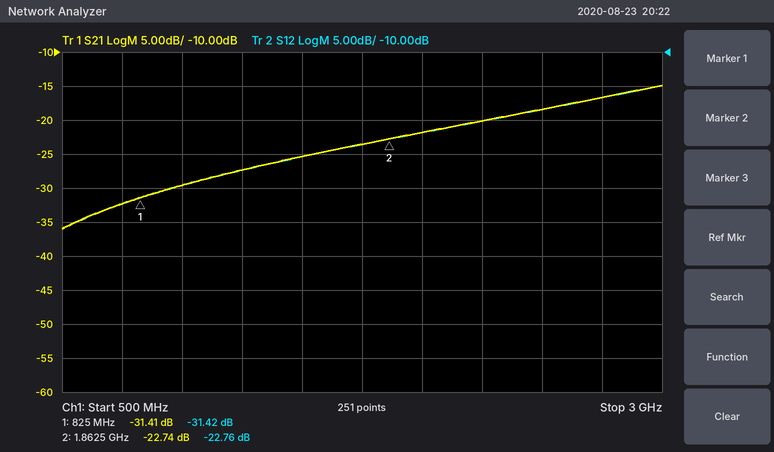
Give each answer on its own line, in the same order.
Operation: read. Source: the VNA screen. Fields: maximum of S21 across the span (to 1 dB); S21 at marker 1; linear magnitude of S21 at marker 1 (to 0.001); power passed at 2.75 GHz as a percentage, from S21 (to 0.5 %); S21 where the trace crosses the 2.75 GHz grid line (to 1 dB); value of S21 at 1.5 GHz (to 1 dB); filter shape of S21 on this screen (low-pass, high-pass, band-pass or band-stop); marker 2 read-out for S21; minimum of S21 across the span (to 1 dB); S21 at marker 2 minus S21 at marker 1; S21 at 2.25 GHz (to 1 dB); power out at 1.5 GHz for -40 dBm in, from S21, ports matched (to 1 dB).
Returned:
-15 dB
-31.41 dB
0.027
2.0 %
-17 dB
-25 dB
high-pass
-22.74 dB
-36 dB
8.67 dB
-20 dB
-65 dBm
